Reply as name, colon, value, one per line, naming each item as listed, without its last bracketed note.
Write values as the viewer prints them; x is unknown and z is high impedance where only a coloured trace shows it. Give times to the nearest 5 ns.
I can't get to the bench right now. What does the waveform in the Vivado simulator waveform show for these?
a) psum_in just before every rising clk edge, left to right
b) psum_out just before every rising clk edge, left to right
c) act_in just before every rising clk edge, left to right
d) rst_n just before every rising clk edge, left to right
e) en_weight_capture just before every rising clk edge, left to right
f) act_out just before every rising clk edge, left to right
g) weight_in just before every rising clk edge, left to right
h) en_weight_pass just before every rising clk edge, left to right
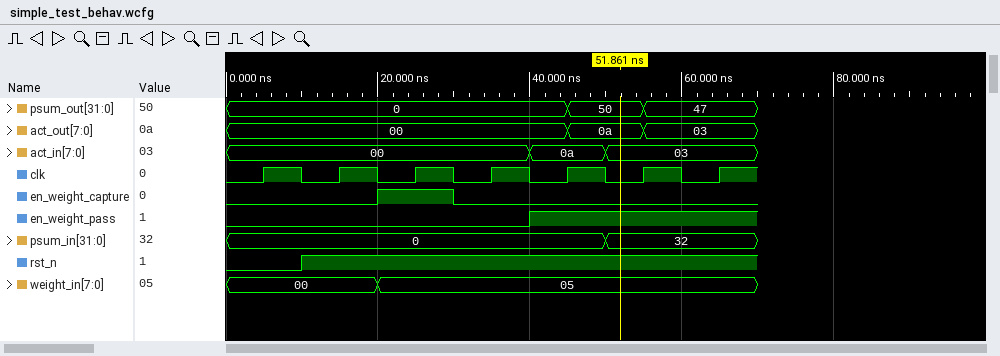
psum_in just before every rising clk edge, left to right: 0, 0, 0, 0, 0, 32, 32
psum_out just before every rising clk edge, left to right: 0, 0, 0, 0, 0, 50, 47
act_in just before every rising clk edge, left to right: 00, 00, 00, 00, 0a, 03, 03
rst_n just before every rising clk edge, left to right: 0 1 1 1 1 1 1
en_weight_capture just before every rising clk edge, left to right: 0 0 1 0 0 0 0
act_out just before every rising clk edge, left to right: 00, 00, 00, 00, 00, 0a, 03
weight_in just before every rising clk edge, left to right: 00, 00, 05, 05, 05, 05, 05
en_weight_pass just before every rising clk edge, left to right: 0 0 0 0 1 1 1
